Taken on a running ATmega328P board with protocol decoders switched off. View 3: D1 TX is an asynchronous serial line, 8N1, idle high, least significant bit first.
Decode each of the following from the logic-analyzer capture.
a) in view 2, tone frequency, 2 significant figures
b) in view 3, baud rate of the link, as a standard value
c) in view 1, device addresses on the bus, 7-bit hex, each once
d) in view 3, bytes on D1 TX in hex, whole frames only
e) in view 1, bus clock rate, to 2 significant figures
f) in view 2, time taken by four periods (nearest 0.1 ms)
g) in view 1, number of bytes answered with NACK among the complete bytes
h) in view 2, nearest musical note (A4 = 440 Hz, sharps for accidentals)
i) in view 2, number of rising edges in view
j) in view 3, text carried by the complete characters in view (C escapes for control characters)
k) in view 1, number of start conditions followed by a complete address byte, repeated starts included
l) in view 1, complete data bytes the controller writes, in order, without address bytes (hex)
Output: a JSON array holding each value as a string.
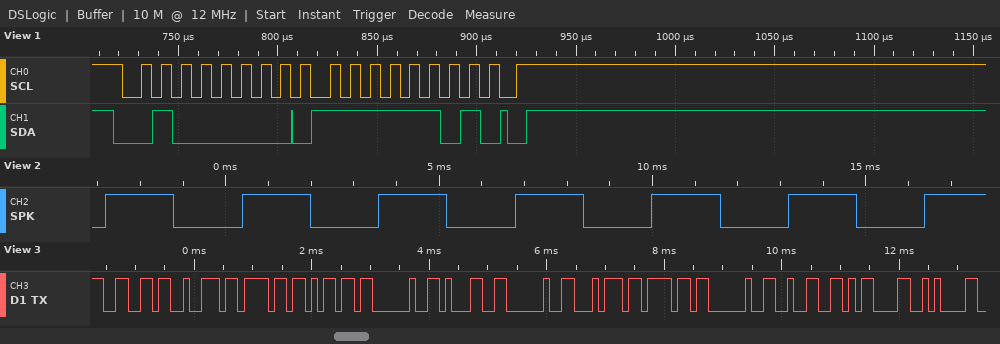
["310 Hz", "9600 baud", "0x20", "0x66 0x72 0x6F 0x6D 0x20 0x31 0x20 0x74 0x6F 0x20 0x32 0x0D 0x0A", "100 kHz", "12.8 ms", "0", "D#4", "7", "\"from 1 to 2\\r\\n\"", "1", "FD"]
